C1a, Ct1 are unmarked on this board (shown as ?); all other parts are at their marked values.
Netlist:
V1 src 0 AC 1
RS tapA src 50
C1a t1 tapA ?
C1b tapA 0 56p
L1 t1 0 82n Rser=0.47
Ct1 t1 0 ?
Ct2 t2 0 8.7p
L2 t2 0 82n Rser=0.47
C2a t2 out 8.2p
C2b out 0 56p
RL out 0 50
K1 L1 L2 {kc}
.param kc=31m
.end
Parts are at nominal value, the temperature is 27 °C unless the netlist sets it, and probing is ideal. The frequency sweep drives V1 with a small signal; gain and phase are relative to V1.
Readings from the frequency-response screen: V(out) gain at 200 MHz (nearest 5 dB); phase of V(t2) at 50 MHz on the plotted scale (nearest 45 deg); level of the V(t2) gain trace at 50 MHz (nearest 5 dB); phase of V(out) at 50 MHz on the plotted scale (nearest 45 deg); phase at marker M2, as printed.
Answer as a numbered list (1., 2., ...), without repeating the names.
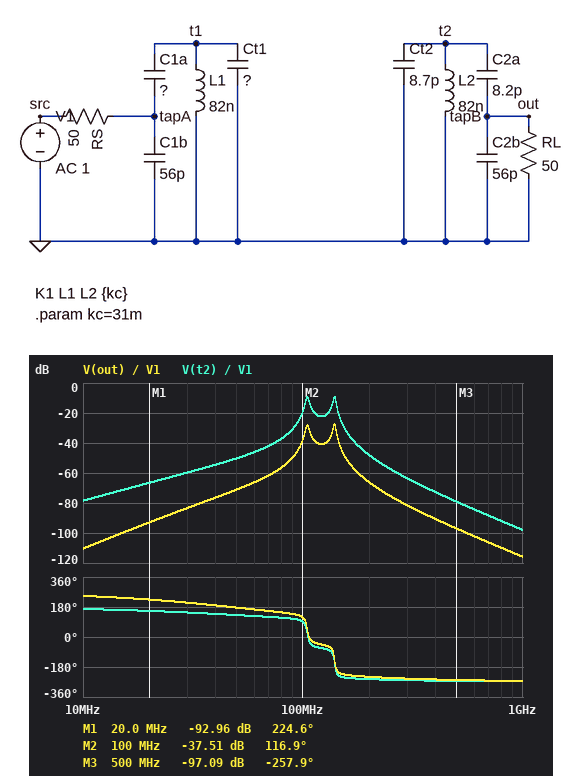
1. -65 dB
2. 135 deg
3. -50 dB
4. 180 deg
5. 116.9 deg
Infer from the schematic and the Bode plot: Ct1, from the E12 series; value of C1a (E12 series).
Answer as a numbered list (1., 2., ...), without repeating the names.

1. 18 pF
2. 12 pF
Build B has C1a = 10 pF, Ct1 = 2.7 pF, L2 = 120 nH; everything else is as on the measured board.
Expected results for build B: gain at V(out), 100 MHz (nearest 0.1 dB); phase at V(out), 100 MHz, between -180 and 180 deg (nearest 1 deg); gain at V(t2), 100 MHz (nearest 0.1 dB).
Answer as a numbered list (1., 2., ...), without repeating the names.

1. -48.0 dB
2. 134 deg
3. -29.1 dB
